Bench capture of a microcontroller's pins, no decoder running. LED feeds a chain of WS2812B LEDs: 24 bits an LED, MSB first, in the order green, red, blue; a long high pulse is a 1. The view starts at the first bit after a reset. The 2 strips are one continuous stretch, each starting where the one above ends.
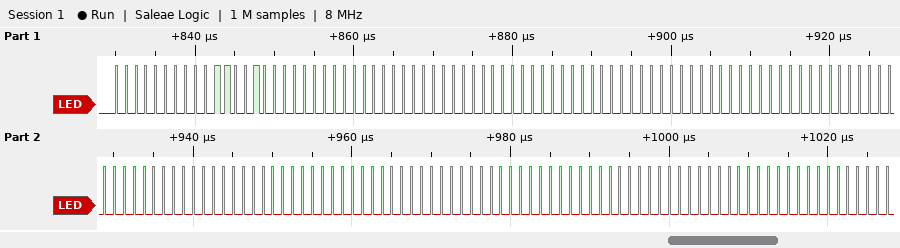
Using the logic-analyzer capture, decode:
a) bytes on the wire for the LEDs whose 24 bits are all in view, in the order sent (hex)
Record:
00 32 00 00 00 00 00 00 00 00 00 00 00 00 00 00 00 00
